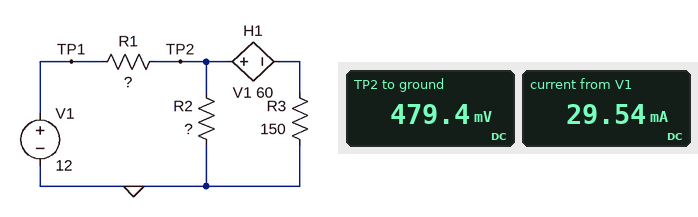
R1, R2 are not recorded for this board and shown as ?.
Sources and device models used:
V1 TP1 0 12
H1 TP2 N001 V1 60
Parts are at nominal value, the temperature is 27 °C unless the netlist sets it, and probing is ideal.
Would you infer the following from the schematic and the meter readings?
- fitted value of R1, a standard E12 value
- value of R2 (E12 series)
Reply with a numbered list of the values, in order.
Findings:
1. 390 Ω
2. 33 Ω
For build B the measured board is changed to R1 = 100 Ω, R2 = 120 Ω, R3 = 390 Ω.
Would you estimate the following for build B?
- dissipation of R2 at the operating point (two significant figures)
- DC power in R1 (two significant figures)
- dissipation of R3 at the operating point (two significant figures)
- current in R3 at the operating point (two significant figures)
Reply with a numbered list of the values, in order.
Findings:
1. 230 mW
2. 460 mW
3. 220 mW
4. 24 mA
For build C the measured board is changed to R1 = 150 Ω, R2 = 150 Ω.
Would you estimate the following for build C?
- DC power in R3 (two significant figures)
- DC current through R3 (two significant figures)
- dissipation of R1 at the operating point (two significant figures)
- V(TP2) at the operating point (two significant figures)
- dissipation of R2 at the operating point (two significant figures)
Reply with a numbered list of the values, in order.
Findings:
1. 280 mW
2. 43 mA
3. 570 mW
4. 2.8 V
5. 51 mW
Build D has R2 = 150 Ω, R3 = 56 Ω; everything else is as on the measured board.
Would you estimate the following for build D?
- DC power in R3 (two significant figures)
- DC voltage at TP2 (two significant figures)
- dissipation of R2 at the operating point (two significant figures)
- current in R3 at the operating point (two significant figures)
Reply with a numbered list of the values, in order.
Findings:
1. 56 mW
2. -90 mV
3. 54 µW
4. 32 mA
